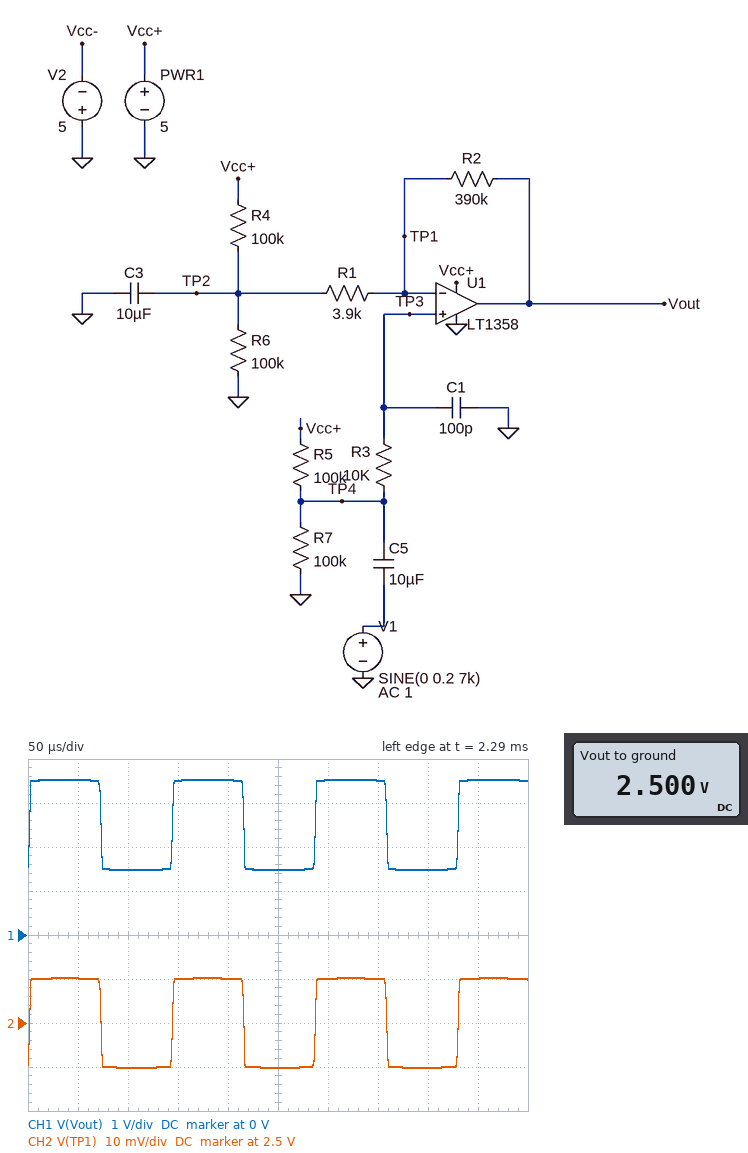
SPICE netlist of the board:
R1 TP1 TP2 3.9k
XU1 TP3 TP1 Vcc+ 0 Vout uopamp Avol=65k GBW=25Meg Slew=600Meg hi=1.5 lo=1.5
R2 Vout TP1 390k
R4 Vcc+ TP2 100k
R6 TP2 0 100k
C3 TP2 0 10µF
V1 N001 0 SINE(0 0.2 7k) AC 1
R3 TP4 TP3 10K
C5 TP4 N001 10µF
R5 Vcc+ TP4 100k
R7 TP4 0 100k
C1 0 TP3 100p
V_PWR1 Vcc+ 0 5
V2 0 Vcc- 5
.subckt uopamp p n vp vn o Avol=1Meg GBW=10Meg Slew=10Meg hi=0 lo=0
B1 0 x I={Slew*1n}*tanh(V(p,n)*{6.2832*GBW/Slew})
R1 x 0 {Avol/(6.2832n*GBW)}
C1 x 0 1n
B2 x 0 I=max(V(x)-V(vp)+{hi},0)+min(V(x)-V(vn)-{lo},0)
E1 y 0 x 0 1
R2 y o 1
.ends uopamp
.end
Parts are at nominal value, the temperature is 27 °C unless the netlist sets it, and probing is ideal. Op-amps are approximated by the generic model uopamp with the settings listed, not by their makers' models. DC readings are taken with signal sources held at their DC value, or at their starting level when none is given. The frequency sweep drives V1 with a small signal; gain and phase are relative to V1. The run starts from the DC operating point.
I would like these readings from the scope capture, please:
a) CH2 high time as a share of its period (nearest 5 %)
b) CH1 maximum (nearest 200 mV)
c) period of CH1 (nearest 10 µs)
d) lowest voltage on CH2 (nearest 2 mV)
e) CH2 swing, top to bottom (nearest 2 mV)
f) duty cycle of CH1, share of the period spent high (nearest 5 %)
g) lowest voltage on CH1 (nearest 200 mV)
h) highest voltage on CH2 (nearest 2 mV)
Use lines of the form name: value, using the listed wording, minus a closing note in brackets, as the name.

CH2 high time as a share of its period: 50 %
CH1 maximum: 3.6 V
period of CH1: 140 µs
lowest voltage on CH2: 2.490 V
CH2 swing, top to bottom: 20 mV
duty cycle of CH1, share of the period spent high: 50 %
lowest voltage on CH1: 1.4 V
highest voltage on CH2: 2.510 V
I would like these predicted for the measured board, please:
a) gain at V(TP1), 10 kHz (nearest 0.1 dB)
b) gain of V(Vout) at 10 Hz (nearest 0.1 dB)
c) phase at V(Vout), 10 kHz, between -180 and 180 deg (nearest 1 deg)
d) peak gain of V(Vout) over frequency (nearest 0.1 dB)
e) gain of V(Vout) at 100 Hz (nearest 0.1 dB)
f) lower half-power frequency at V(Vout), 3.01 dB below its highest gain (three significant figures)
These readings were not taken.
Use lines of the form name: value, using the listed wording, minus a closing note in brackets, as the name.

gain at V(TP1), 10 kHz: 0 dB
gain of V(Vout) at 10 Hz: 39.3 dB
phase at V(Vout), 10 kHz, between -180 and 180 deg: -6 deg
peak gain of V(Vout) over frequency: 40.1 dB
gain of V(Vout) at 100 Hz: 40.1 dB
lower half-power frequency at V(Vout), 3.01 dB below its highest gain: 4.39 Hz
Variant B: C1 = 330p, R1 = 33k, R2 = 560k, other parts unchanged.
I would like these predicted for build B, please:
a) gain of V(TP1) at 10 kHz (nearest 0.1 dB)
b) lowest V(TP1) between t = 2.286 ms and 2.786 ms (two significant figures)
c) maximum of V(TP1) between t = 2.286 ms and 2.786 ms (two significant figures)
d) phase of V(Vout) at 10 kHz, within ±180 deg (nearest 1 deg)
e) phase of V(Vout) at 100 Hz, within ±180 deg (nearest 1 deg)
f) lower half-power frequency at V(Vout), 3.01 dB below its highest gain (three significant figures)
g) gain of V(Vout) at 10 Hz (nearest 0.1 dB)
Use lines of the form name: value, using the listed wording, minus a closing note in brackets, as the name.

gain of V(TP1) at 10 kHz: -0.2 dB
lowest V(TP1) between t = 2.286 ms and 2.786 ms: 2.4 V
maximum of V(TP1) between t = 2.286 ms and 2.786 ms: 2.6 V
phase of V(Vout) at 10 kHz, within ±180 deg: -12 deg
phase of V(Vout) at 100 Hz, within ±180 deg: 0 deg
lower half-power frequency at V(Vout), 3.01 dB below its highest gain: 781 mHz
gain of V(Vout) at 10 Hz: 25.1 dB
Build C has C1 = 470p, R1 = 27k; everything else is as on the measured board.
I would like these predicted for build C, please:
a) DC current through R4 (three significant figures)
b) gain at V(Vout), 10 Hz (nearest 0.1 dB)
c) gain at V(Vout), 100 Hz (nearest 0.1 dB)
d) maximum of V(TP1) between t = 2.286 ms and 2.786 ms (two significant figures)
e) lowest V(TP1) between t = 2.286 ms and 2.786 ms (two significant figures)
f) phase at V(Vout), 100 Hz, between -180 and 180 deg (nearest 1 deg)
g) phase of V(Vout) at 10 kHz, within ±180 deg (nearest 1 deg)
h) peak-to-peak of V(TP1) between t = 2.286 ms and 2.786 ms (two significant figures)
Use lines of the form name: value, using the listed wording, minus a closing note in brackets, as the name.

DC current through R4: 25.0 µA
gain at V(Vout), 10 Hz: 23.7 dB
gain at V(Vout), 100 Hz: 23.8 dB
maximum of V(TP1) between t = 2.286 ms and 2.786 ms: 2.6 V
lowest V(TP1) between t = 2.286 ms and 2.786 ms: 2.4 V
phase at V(Vout), 100 Hz, between -180 and 180 deg: 0 deg
phase of V(Vout) at 10 kHz, within ±180 deg: -17 deg
peak-to-peak of V(TP1) between t = 2.286 ms and 2.786 ms: 130 mV
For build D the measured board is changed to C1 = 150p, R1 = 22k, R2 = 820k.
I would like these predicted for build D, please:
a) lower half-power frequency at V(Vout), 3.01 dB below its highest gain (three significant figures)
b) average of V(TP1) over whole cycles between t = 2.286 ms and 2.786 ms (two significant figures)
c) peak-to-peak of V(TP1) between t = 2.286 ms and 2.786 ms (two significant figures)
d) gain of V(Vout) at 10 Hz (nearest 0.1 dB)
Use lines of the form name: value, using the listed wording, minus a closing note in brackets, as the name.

lower half-power frequency at V(Vout), 3.01 dB below its highest gain: 1.03 Hz
average of V(TP1) over whole cycles between t = 2.286 ms and 2.786 ms: 2.5 V
peak-to-peak of V(TP1) between t = 2.286 ms and 2.786 ms: 54 mV
gain of V(Vout) at 10 Hz: 31.6 dB
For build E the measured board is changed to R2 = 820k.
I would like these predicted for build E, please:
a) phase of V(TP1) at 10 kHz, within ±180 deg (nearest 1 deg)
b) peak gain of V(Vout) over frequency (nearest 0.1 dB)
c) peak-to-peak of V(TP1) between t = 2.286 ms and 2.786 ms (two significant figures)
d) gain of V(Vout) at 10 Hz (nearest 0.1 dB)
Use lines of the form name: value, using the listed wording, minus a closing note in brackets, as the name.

phase of V(TP1) at 10 kHz, within ±180 deg: -8 deg
peak gain of V(Vout) over frequency: 46.5 dB
peak-to-peak of V(TP1) between t = 2.286 ms and 2.786 ms: 9.8 mV
gain of V(Vout) at 10 Hz: 45.7 dB
